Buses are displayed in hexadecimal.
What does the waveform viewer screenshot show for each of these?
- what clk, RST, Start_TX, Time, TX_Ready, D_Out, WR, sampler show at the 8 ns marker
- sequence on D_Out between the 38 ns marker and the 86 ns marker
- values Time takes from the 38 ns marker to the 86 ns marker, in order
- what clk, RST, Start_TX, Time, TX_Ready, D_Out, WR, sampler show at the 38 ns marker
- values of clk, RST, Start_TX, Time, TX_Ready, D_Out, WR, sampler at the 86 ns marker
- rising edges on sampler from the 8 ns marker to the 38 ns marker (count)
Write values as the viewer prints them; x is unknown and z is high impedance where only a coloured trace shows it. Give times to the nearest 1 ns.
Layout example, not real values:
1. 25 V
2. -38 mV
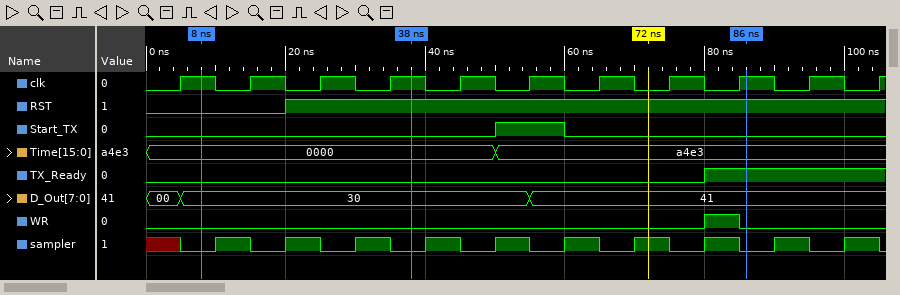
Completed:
1. clk=1, RST=0, Start_TX=0, Time=0000, TX_Ready=0, D_Out=30, WR=0, sampler=0
2. 30, 41
3. 0000, a4e3
4. clk=1, RST=1, Start_TX=0, Time=0000, TX_Ready=0, D_Out=30, WR=0, sampler=0
5. clk=1, RST=1, Start_TX=0, Time=a4e3, TX_Ready=1, D_Out=41, WR=0, sampler=0
6. 3
